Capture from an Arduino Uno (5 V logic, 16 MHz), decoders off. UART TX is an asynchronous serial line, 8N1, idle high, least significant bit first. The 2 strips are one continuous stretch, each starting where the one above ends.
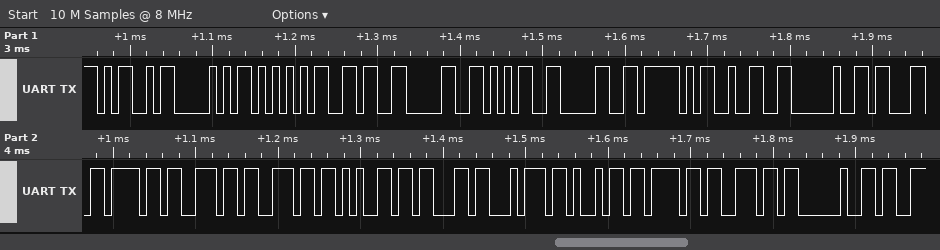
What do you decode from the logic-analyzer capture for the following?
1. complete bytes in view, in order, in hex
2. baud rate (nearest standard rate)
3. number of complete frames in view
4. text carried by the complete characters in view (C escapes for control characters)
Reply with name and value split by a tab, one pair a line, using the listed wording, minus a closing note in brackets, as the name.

complete bytes in view, in order, in hex	4D 50 55 36 30 35 30 5F 32 20 63 6F 6E 6E 65 63 74 69 6F 6E 20
baud rate	115200 baud
number of complete frames in view	21
text carried by the complete characters in view	"MPU6050_2 connection "
